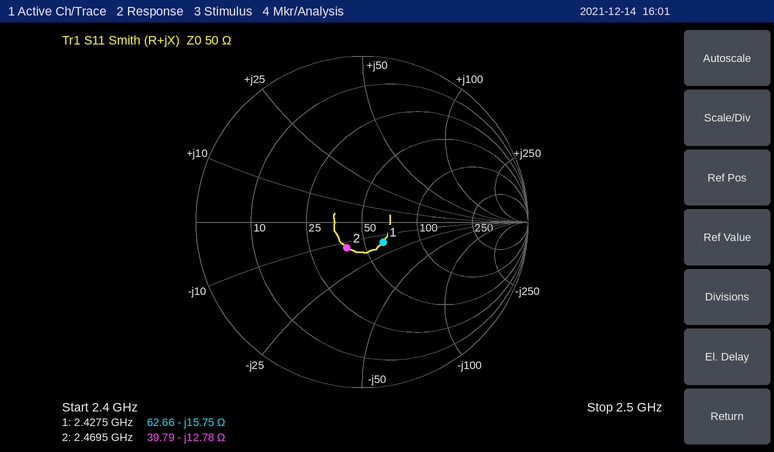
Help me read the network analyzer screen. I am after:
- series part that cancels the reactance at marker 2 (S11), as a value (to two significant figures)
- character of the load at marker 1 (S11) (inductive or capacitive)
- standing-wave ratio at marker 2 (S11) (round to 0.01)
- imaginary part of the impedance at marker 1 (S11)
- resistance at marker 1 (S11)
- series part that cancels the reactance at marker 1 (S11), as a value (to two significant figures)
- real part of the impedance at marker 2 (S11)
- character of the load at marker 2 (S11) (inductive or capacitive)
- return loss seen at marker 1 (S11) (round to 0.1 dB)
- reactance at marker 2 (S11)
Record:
820 pH
capacitive
1.44
-15.75 Ω
62.66 Ω
1.0 nH
39.79 Ω
capacitive
15.0 dB
-12.78 Ω
